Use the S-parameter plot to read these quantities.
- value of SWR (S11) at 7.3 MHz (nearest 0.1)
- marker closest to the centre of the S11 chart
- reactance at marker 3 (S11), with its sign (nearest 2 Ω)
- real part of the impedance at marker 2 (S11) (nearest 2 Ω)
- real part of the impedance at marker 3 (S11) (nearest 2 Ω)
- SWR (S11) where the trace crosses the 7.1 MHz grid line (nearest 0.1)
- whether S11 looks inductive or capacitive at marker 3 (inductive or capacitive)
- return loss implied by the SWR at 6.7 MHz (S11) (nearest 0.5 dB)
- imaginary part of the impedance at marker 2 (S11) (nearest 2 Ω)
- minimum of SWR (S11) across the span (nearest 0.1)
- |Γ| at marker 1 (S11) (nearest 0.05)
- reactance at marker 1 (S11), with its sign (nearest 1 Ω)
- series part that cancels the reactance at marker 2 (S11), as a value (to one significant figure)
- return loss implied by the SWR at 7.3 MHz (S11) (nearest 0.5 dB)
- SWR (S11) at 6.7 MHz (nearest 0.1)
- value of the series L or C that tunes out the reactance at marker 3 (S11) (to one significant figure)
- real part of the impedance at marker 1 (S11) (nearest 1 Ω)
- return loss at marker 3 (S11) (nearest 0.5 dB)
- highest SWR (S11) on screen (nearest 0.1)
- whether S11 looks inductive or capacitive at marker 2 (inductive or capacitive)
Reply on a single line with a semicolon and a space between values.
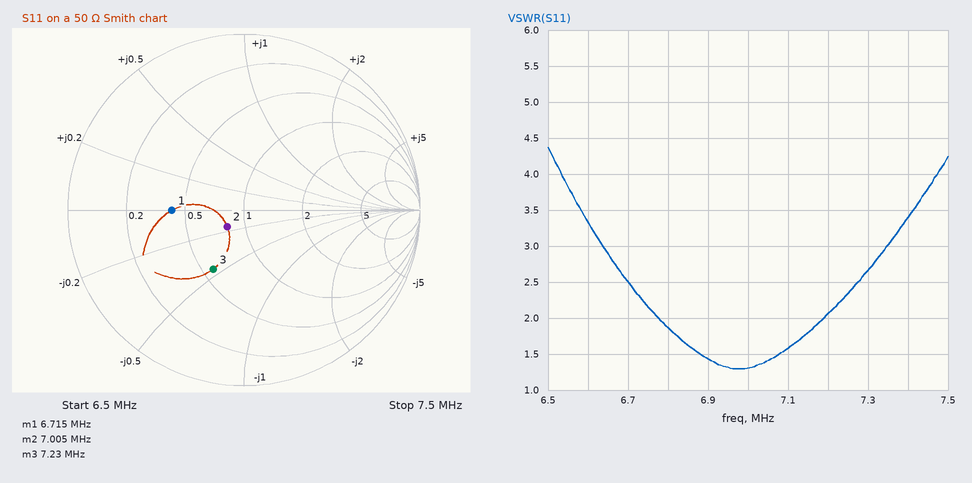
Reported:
2.7; marker 2; -22 Ω; 40 Ω; 28 Ω; 1.6; capacitive; 7.5 dB; -8 Ω; 1.3; 0.40; 0 Ω; 200 nH; 7.0 dB; 2.5; 500 nH; 21 Ω; 8.5 dB; 4.4; capacitive
